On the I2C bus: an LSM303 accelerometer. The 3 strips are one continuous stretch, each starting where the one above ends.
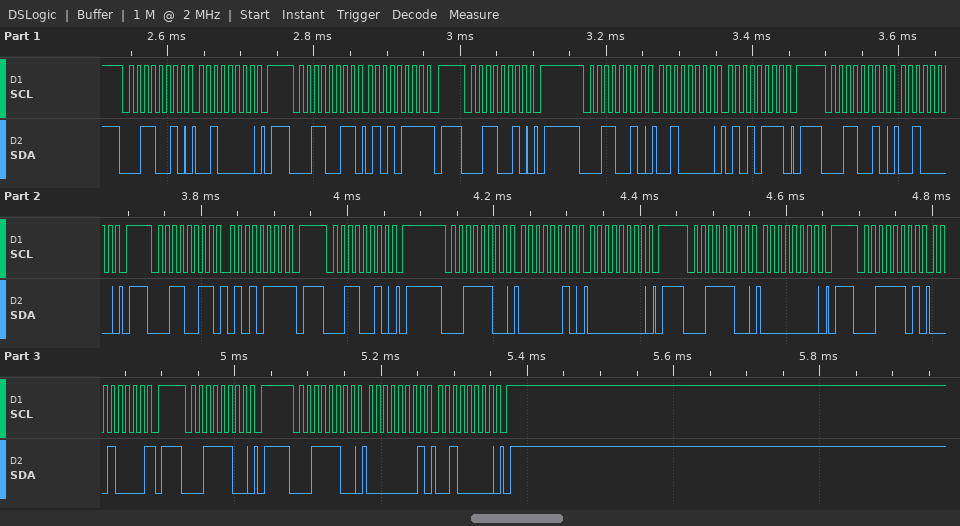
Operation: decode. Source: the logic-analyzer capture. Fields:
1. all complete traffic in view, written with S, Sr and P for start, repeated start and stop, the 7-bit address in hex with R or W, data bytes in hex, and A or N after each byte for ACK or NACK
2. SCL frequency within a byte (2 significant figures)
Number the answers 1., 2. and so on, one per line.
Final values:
1. S 19W A 20 A P S 19R A 57 N P S 19W A P S 19W A 20 A 57 A P S 19W A 20 A P S 19R A 57 N P S 19W A P S 1EW A 02 A 00 A P S 1EW A 00 A P S 1ER A 10 N P S 1EW A P S 1EW A 01 A 20 A P
2. 100 kHz
